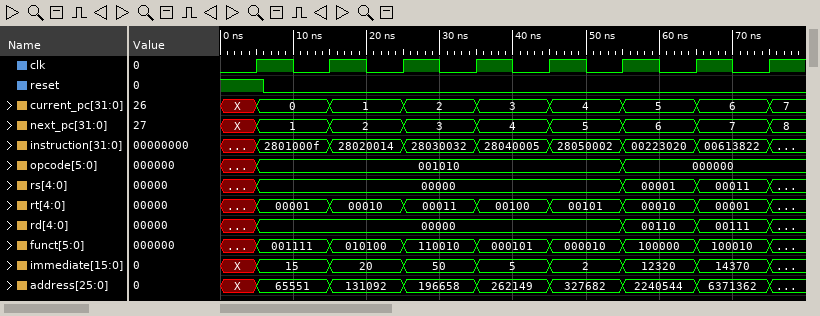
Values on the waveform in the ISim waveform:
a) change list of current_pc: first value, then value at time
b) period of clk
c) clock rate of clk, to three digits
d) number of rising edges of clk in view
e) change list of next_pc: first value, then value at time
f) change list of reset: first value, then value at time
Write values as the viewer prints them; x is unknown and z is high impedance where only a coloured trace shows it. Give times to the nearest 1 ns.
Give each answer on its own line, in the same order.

X, 0 at 5 ns, 1 at 15 ns, 2 at 25 ns, 3 at 35 ns, 4 at 45 ns, 5 at 55 ns, 6 at 65 ns, 7 at 75 ns
10 ns
100 MHz
8
X, 1 at 5 ns, 2 at 15 ns, 3 at 25 ns, 4 at 35 ns, 5 at 45 ns, 6 at 55 ns, 7 at 65 ns, 8 at 75 ns
1, 0 at 6 ns
